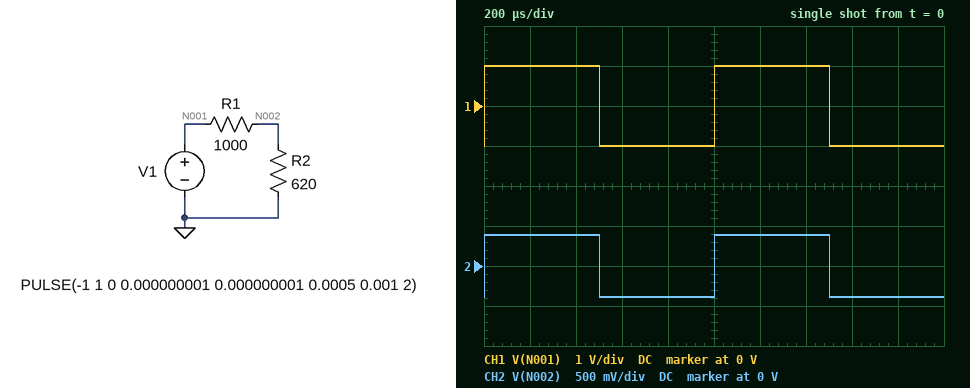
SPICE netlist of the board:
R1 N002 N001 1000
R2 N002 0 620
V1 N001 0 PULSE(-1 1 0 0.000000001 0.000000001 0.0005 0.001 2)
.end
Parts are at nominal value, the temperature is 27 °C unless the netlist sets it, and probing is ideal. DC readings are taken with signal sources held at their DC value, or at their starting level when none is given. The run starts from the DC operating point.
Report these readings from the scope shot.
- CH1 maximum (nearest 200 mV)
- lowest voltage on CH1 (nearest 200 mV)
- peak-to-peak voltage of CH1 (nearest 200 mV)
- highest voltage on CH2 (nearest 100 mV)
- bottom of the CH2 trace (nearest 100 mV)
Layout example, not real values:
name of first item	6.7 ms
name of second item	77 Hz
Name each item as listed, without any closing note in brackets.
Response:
CH1 maximum	1.0 V
lowest voltage on CH1	-1.0 V
peak-to-peak voltage of CH1	2.0 V
highest voltage on CH2	400 mV
bottom of the CH2 trace	-400 mV
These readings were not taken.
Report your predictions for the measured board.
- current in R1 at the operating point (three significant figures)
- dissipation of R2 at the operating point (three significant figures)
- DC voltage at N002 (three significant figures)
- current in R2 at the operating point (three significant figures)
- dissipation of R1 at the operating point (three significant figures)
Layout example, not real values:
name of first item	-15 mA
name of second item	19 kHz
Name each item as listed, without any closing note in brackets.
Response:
current in R1 at the operating point	617 µA
dissipation of R2 at the operating point	236 µW
DC voltage at N002	-383 mV
current in R2 at the operating point	617 µA
dissipation of R1 at the operating point	381 µW
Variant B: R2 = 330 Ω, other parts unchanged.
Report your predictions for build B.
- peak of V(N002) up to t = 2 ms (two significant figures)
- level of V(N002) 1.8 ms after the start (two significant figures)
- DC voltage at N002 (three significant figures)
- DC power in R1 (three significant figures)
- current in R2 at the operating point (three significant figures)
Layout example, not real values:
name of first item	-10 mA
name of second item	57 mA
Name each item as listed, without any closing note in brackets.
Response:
peak of V(N002) up to t = 2 ms	250 mV
level of V(N002) 1.8 ms after the start	-250 mV
DC voltage at N002	-248 mV
DC power in R1	565 µW
current in R2 at the operating point	752 µA
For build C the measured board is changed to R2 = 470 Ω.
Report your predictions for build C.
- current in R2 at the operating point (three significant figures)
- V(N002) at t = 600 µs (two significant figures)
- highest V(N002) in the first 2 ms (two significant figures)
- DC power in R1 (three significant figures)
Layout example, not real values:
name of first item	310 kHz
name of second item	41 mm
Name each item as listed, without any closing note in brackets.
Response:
current in R2 at the operating point	680 µA
V(N002) at t = 600 µs	-320 mV
highest V(N002) in the first 2 ms	320 mV
DC power in R1	463 µW
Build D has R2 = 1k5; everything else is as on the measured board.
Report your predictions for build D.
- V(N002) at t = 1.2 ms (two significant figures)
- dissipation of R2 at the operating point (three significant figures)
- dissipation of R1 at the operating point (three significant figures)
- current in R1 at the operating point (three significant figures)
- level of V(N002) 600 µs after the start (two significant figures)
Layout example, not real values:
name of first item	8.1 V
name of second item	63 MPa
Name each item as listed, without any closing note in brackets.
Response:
V(N002) at t = 1.2 ms	600 mV
dissipation of R2 at the operating point	240 µW
dissipation of R1 at the operating point	160 µW
current in R1 at the operating point	400 µA
level of V(N002) 600 µs after the start	-600 mV
